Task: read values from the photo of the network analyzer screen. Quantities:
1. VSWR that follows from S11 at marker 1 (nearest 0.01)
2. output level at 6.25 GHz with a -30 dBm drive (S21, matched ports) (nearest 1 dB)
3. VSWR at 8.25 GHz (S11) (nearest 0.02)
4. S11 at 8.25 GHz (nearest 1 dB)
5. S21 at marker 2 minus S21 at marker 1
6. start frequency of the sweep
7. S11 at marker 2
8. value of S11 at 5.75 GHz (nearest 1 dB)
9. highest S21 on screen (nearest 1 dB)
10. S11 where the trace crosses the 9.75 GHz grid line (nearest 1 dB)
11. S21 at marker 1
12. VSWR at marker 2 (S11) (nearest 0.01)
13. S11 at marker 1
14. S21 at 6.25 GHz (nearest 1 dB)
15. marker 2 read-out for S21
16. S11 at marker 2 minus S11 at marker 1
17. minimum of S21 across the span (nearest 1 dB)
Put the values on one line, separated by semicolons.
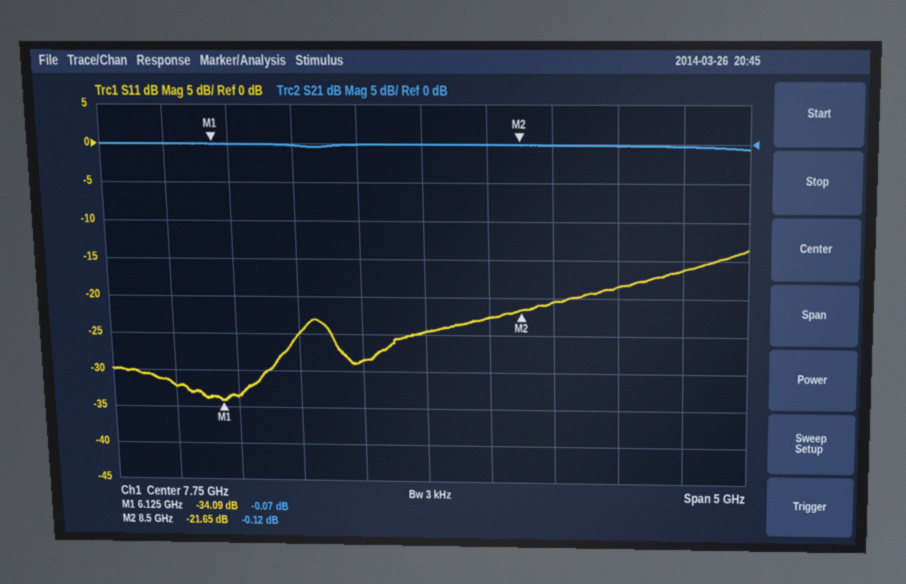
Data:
1.04; -30 dBm; 1.16; -23 dB; -0.05 dB; 5.25 GHz; -21.65 dB; -32 dB; 0 dB; -16 dB; -0.07 dB; 1.18; -34.09 dB; 0 dB; -0.12 dB; 12.44 dB; -1 dB
